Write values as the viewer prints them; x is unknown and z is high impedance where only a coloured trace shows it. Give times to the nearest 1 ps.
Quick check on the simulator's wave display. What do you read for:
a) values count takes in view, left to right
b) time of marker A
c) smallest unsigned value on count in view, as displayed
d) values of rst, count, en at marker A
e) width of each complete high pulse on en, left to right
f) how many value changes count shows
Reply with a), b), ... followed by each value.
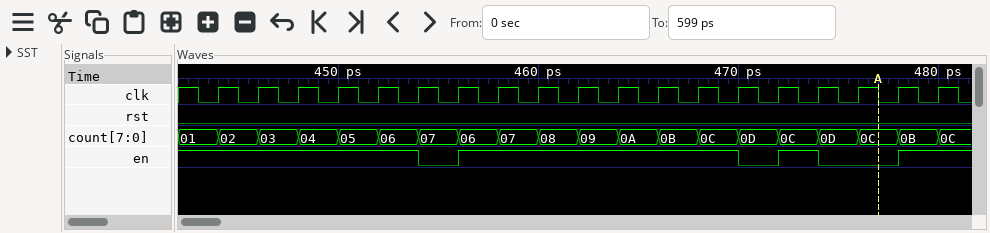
a) 01, 02, 03, 04, 05, 06, 07, 06, 07, 08, 09, 0A, 0B, 0C, 0D, 0C, 0D, 0C, 0B, 0C
b) 477 ps
c) 01
d) rst=0, count=0C, en=0
e) 14 ps, 2 ps
f) 19
